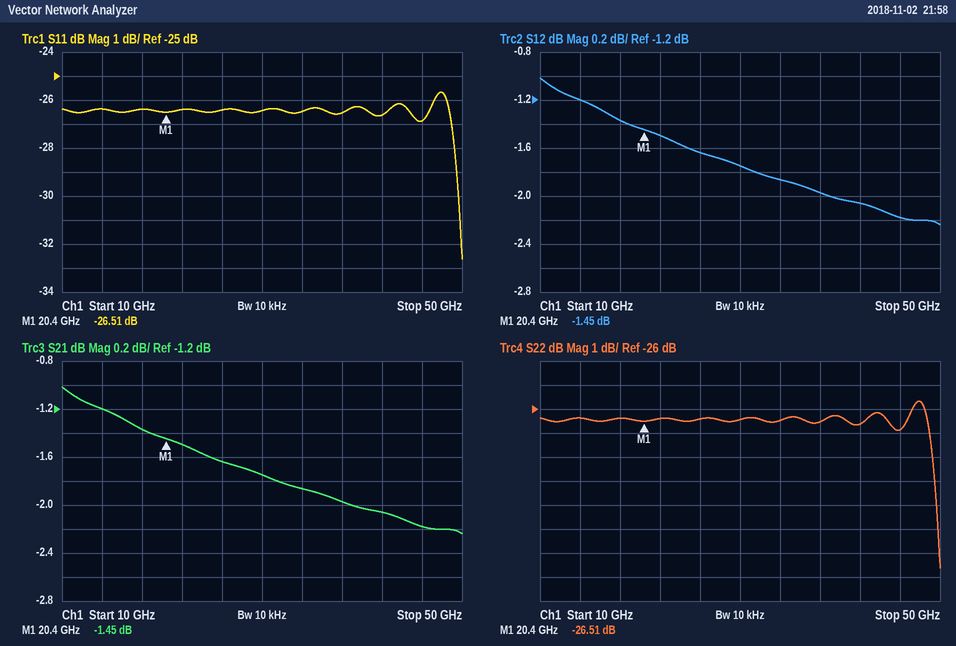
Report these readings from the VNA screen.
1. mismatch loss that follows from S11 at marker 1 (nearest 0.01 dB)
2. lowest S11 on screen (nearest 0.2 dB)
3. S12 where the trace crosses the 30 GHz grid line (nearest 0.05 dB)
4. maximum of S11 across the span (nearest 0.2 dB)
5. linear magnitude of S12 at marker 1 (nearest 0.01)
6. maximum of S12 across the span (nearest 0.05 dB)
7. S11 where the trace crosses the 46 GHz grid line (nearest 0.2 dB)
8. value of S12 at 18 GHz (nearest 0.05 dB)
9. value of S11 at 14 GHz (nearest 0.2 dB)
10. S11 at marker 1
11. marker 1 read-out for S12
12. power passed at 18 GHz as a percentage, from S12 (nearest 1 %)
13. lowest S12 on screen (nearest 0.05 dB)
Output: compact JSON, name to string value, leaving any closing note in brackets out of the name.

{"mismatch loss that follows from S11 at marker 1": "0.01 dB", "lowest S11 on screen": "-32.6 dB", "S12 where the trace crosses the 30 GHz grid line": "-1.75 dB", "maximum of S11 across the span": "-25.6 dB", "linear magnitude of S12 at marker 1": "0.85", "maximum of S12 across the span": "-1.00 dB", "S11 where the trace crosses the 46 GHz grid line": "-26.8 dB", "value of S12 at 18 GHz": "-1.35 dB", "value of S11 at 14 GHz": "-26.4 dB", "S11 at marker 1": "-26.51 dB", "marker 1 read-out for S12": "-1.45 dB", "power passed at 18 GHz as a percentage, from S12": "73 %", "lowest S12 on screen": "-2.25 dB"}
